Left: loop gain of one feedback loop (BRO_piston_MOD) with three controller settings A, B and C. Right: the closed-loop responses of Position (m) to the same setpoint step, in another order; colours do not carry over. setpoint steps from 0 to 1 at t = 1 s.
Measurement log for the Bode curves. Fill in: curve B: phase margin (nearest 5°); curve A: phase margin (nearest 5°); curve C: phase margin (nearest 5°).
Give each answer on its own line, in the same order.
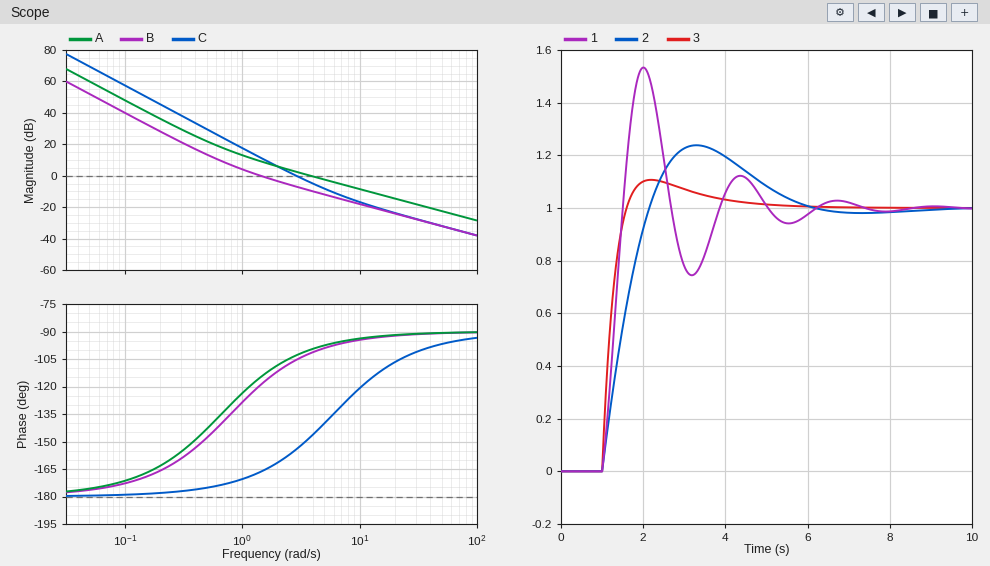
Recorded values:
60°
80°
25°
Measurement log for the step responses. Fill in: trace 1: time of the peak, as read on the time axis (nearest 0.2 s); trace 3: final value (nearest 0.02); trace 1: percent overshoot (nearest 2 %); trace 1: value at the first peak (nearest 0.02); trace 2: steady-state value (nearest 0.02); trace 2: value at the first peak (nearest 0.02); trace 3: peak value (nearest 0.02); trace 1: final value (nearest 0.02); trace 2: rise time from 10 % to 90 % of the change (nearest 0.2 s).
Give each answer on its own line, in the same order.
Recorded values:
2.0 s
1.00
54 %
1.54
1.00
1.24
1.10
1.00
0.8 s
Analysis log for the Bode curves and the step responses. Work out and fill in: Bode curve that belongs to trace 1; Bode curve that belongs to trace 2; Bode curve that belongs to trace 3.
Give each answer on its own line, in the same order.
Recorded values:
C
B
A
